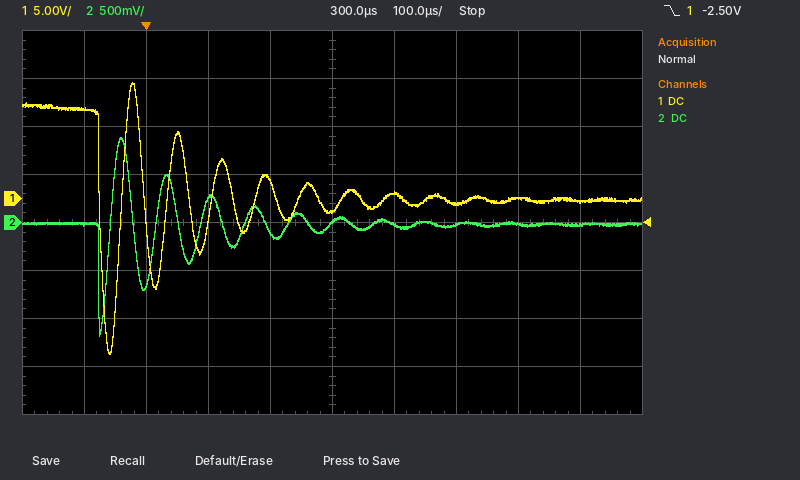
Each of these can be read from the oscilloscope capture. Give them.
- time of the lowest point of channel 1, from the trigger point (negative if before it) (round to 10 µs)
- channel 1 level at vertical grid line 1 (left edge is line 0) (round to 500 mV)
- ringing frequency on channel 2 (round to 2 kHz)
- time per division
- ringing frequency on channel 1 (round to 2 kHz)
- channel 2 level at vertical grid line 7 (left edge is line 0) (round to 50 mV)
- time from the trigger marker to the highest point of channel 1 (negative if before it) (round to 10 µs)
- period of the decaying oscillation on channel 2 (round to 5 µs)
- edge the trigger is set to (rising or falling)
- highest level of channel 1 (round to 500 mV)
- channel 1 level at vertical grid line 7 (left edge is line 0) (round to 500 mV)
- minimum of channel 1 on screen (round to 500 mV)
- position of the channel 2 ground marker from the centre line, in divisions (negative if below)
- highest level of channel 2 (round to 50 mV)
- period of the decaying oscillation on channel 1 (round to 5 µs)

-60 µs
9.5 V
14 kHz
100 µs
14 kHz
0 mV
-20 µs
70 µs
falling
12.0 V
-500 mV
-16.0 V
0.0 div
900 mV
70 µs
